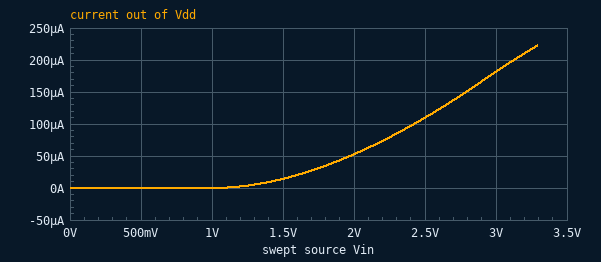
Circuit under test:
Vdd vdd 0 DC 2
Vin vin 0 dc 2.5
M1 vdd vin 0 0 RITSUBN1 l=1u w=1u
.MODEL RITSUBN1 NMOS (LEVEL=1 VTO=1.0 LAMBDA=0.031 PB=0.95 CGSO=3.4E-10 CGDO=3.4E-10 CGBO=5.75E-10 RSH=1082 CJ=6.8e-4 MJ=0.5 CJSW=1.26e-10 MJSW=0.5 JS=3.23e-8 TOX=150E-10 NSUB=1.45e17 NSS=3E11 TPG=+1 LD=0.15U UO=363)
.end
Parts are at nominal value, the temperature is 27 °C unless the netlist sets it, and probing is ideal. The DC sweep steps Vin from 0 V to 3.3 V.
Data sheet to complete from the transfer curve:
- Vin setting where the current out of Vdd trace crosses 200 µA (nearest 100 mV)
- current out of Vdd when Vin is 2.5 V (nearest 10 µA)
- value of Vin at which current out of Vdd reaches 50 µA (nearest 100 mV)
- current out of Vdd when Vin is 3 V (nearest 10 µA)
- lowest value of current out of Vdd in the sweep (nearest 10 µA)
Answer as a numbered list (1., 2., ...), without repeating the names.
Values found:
1. 3.1 V
2. 110 µA
3. 2.0 V
4. 180 µA
5. 0 A
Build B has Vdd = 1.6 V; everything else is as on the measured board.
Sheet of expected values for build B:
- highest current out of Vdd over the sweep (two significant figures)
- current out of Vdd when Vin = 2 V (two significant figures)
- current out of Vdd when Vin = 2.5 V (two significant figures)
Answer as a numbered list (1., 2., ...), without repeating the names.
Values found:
1. 200 µA
2. 52 µA
3. 110 µA
